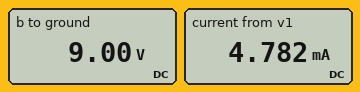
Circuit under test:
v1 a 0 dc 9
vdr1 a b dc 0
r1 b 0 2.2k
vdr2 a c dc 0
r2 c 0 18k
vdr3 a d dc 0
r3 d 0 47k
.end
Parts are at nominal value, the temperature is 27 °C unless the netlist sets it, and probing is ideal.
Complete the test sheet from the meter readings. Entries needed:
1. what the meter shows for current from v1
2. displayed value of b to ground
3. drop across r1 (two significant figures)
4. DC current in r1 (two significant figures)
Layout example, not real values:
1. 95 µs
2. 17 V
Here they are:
1. 4.782 mA
2. 9.00 V
3. 9.0 V
4. 4.1 mA
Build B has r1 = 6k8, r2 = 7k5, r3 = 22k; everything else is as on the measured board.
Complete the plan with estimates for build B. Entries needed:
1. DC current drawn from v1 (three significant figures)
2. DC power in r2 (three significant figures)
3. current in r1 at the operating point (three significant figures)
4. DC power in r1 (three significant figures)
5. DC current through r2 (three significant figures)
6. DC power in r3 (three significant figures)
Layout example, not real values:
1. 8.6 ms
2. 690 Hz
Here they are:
1. 2.93 mA
2. 10.8 mW
3. 1.32 mA
4. 11.9 mW
5. 1.20 mA
6. 3.68 mW
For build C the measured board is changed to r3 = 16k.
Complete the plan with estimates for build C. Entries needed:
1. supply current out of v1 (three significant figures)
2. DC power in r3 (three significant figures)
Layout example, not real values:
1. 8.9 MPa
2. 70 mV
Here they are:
1. 5.15 mA
2. 5.06 mW
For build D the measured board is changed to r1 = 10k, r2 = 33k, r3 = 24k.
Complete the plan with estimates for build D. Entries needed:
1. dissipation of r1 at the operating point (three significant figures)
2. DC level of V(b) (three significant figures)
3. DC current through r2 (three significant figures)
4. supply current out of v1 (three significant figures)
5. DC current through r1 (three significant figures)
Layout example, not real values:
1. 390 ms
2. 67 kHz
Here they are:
1. 8.10 mW
2. 9.00 V
3. 273 µA
4. 1.55 mA
5. 900 µA
